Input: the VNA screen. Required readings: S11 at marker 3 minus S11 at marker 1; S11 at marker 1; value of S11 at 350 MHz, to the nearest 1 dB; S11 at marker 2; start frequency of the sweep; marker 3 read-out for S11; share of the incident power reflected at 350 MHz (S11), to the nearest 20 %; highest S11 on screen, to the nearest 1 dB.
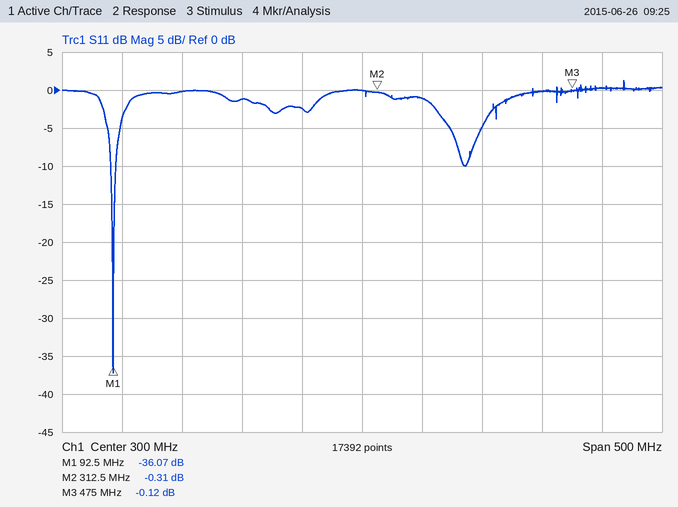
35.95 dB
-36.07 dB
-1 dB
-0.31 dB
50 MHz
-0.12 dB
80 %
1 dB
